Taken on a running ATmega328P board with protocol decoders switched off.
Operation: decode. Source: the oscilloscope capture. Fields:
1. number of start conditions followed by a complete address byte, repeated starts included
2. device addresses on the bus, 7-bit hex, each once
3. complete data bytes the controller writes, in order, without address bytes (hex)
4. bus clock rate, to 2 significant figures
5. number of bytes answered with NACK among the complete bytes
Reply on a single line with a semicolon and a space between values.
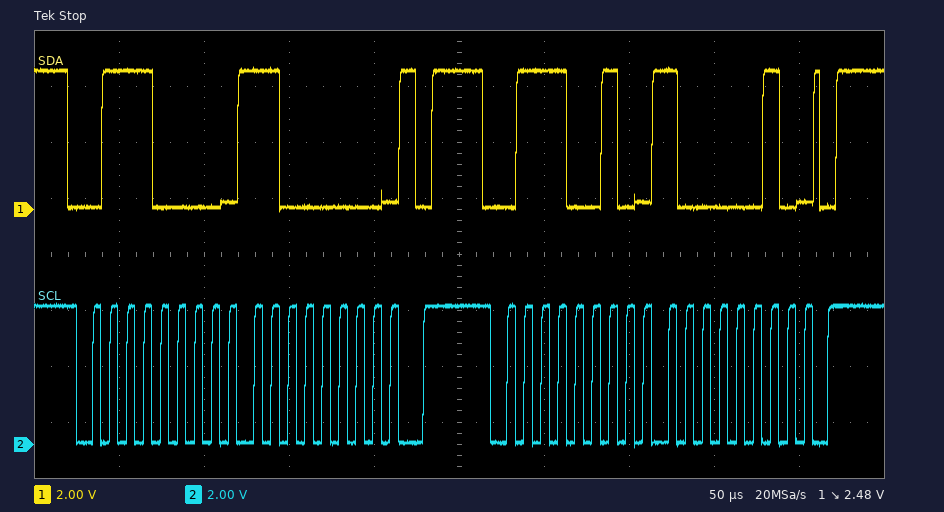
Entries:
2; 0x38 0x39; C0 82; 100 kHz; 0
